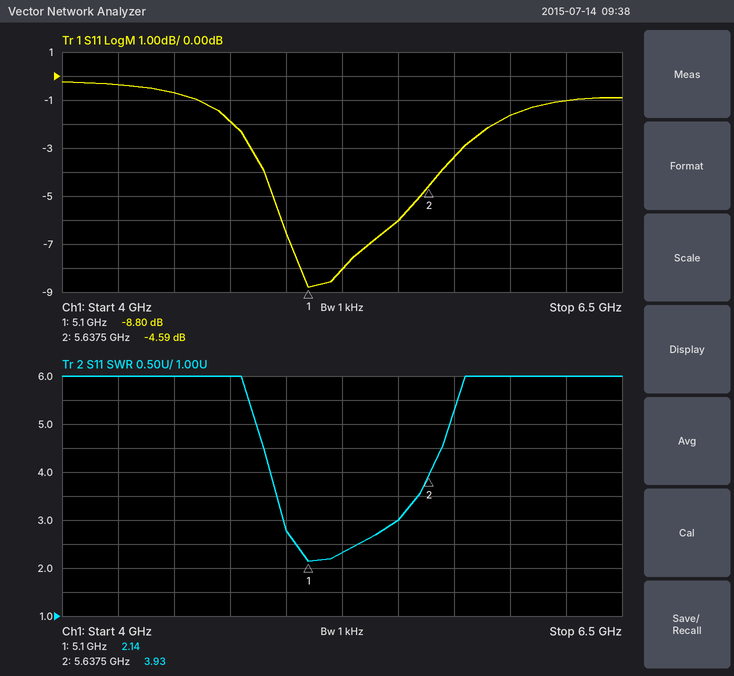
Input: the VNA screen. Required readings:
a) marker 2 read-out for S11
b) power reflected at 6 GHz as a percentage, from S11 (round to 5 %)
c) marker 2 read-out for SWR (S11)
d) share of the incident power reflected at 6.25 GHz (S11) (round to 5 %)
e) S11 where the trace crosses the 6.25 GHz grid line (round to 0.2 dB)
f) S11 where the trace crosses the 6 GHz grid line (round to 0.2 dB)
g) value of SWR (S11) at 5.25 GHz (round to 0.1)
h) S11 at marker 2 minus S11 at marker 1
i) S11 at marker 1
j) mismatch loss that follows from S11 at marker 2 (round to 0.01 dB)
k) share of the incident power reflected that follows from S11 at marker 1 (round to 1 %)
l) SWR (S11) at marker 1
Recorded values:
-4.59 dB
70 %
3.93
80 %
-1.0 dB
-1.6 dB
2.3
4.21 dB
-8.80 dB
1.85 dB
13 %
2.14
